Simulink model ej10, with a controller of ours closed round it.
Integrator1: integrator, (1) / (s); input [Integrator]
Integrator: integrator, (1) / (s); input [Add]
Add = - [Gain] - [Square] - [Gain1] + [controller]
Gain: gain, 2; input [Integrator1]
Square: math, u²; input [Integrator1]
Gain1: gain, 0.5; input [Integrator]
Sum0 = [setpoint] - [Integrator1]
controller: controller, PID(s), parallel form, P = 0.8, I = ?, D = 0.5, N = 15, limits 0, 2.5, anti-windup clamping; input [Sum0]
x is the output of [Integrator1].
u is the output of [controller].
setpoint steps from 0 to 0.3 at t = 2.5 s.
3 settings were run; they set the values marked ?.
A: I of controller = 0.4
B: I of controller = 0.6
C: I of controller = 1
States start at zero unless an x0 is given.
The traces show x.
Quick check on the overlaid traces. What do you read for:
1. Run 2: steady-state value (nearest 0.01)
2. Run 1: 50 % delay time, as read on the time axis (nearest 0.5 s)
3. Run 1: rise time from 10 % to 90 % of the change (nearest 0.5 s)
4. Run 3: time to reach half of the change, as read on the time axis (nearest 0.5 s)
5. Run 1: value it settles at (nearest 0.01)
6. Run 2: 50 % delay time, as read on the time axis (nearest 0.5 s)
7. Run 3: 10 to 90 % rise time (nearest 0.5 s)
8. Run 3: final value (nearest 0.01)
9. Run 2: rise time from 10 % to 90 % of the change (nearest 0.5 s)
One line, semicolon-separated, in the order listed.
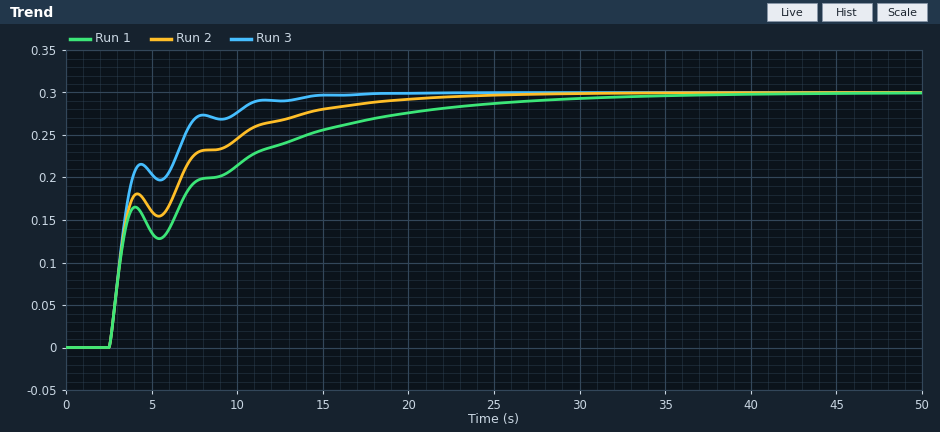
0.30; 3.5 s; 15.5 s; 3.5 s; 0.30; 3.5 s; 5.0 s; 0.30; 10.5 s
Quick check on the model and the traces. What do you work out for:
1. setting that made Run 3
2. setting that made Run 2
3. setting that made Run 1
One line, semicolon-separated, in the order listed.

C; B; A
